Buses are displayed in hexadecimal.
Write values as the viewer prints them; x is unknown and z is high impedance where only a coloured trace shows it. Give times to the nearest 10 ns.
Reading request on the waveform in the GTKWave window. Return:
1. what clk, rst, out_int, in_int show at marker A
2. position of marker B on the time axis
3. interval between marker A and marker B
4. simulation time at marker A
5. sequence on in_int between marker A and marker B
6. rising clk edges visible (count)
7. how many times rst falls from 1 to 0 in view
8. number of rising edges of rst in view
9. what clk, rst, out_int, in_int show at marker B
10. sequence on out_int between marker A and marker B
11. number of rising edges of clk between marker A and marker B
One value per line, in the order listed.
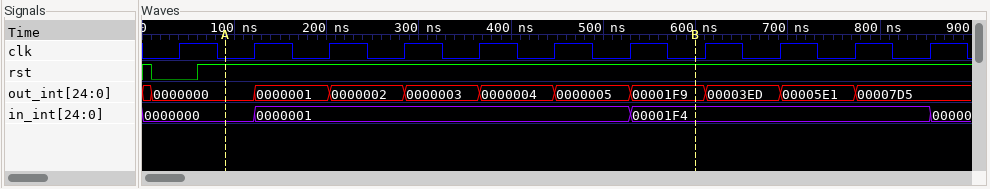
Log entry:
clk=0, rst=1, out_int=0000000, in_int=0000000
600 ns
510 ns
90 ns
0000000, 0000001, 00001F4
11
1
1
clk=0, rst=1, out_int=00001F9, in_int=00001F4
0000000, 0000001, 0000002, 0000003, 0000004, 0000005, 00001F9
6
